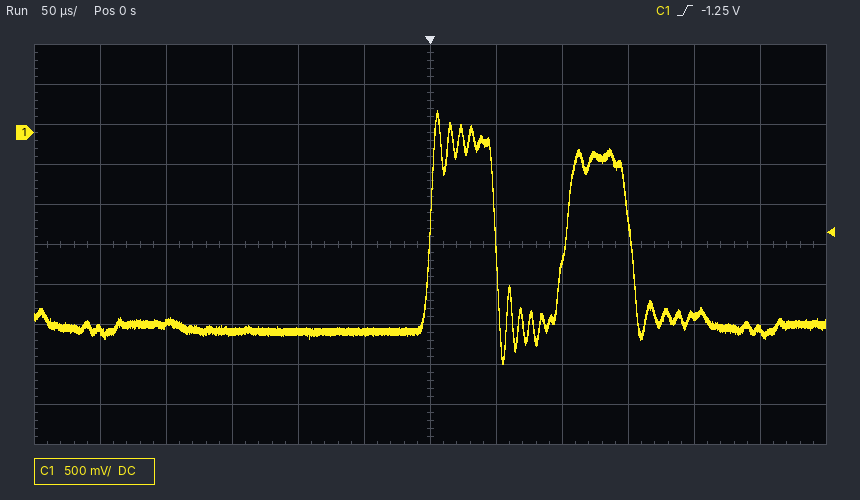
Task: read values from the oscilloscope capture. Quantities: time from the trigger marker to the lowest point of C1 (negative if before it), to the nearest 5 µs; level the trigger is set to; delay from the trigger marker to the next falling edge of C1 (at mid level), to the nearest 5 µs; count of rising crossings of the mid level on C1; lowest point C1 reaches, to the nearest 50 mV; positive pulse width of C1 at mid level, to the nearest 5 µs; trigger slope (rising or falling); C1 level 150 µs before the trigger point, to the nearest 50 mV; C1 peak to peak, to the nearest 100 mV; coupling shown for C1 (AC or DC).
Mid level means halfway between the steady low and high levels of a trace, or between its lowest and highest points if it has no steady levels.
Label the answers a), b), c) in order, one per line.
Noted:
a) +55 µs
b) -1.25 V
c) 50 µs
d) 2
e) -2.90 V
f) 50 µs
g) rising
h) -2.50 V
i) 3.20 V
j) DC
